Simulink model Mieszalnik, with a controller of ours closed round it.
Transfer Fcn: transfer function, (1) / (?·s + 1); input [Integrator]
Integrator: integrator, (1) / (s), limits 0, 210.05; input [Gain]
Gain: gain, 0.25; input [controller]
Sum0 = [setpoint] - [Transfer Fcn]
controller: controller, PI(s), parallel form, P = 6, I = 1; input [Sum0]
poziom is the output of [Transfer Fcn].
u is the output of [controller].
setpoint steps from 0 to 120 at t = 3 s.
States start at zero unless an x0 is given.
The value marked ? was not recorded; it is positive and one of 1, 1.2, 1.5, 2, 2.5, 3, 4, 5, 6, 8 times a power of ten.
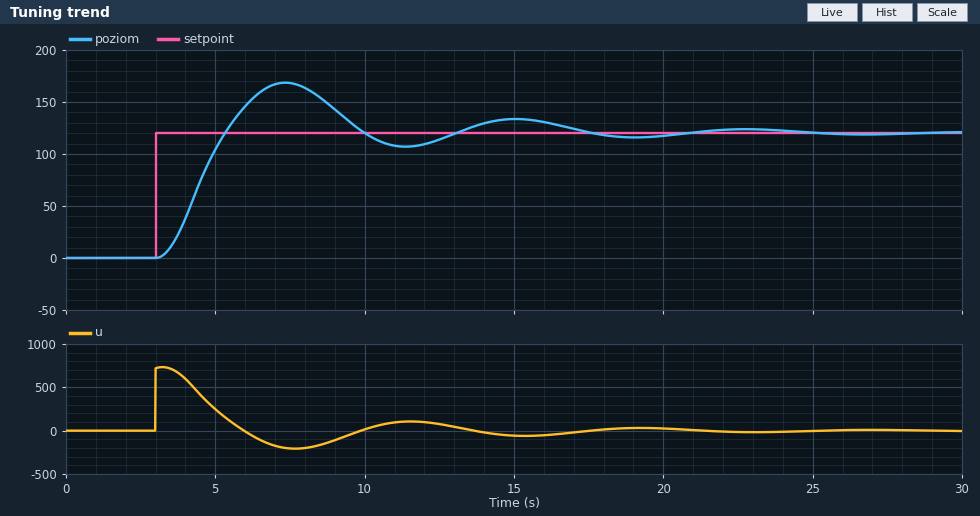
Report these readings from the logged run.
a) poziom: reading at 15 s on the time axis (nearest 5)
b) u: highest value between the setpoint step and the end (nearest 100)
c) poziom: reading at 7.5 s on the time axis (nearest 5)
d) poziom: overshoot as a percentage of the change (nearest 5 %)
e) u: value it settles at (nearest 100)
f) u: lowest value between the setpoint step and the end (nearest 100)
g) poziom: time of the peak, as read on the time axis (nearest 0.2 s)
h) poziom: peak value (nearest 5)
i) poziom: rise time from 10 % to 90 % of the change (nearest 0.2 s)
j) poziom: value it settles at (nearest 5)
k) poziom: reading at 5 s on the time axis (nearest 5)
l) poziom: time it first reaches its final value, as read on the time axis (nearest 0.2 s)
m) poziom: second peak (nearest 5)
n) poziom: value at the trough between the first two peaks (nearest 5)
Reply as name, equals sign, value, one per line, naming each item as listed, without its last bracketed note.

poziom: reading at 15 s on the time axis = 135
u: highest value between the setpoint step and the end = 700
poziom: reading at 7.5 s on the time axis = 170
poziom: overshoot as a percentage of the change = 40 %
u: value it settles at = 0
u: lowest value between the setpoint step and the end = -200
poziom: time of the peak, as read on the time axis = 7.4 s
poziom: peak value = 170
poziom: rise time from 10 % to 90 % of the change = 1.6 s
poziom: value it settles at = 120
poziom: reading at 5 s on the time axis = 105
poziom: time it first reaches its final value, as read on the time axis = 5.4 s
poziom: second peak = 135
poziom: value at the trough between the first two peaks = 105
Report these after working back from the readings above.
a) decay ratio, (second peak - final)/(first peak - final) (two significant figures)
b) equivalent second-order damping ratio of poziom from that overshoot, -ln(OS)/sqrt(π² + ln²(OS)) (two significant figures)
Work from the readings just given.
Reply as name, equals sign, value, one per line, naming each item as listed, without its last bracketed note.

decay ratio, (second peak - final)/(first peak - final) = 0.30
equivalent second-order damping ratio of poziom from that overshoot, -ln(OS)/sqrt(π² + ln²(OS)) = 0.28
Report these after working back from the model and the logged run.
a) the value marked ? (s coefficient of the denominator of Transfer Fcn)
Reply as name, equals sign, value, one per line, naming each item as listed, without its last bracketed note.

the value marked ? = 2
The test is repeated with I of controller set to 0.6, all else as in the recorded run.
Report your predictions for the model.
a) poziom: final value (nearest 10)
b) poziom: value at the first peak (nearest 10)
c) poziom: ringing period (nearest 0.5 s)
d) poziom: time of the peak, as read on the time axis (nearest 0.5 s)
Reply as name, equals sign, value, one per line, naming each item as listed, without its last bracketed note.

poziom: final value = 120
poziom: value at the first peak = 160
poziom: ringing period = 7.5 s
poziom: time of the peak, as read on the time axis = 7.0 s
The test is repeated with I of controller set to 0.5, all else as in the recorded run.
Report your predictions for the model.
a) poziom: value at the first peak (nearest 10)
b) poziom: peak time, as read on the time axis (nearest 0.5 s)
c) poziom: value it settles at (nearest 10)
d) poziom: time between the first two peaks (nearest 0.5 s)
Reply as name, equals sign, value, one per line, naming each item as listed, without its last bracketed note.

poziom: value at the first peak = 160
poziom: peak time, as read on the time axis = 7.0 s
poziom: value it settles at = 120
poziom: time between the first two peaks = 7.5 s
